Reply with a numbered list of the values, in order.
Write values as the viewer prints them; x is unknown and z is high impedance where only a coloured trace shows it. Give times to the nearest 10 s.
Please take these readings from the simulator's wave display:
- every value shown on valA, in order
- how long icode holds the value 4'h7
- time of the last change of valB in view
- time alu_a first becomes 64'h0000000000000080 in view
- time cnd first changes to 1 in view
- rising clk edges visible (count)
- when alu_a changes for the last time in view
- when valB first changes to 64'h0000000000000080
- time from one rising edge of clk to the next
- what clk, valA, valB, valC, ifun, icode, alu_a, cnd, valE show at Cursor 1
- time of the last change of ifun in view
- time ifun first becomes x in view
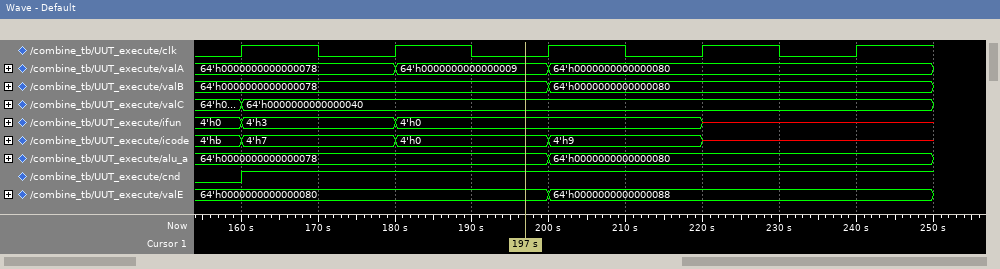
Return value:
1. 64'h0000000000000078, 64'h0000000000000009, 64'h0000000000000080
2. 20 s
3. 200 s
4. 200 s
5. 160 s
6. 5
7. 200 s
8. 200 s
9. 20 s
10. clk=0, valA=64'h0000000000000009, valB=64'h0000000000000078, valC=64'h0000000000000040, ifun=4'h0, icode=4'h0, alu_a=64'h0000000000000078, cnd=1, valE=64'h0000000000000080
11. 220 s
12. 220 s
